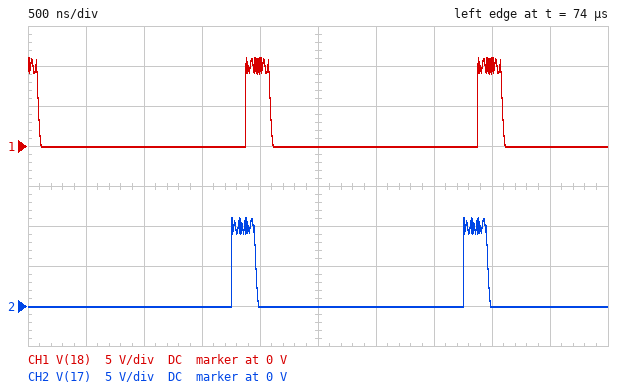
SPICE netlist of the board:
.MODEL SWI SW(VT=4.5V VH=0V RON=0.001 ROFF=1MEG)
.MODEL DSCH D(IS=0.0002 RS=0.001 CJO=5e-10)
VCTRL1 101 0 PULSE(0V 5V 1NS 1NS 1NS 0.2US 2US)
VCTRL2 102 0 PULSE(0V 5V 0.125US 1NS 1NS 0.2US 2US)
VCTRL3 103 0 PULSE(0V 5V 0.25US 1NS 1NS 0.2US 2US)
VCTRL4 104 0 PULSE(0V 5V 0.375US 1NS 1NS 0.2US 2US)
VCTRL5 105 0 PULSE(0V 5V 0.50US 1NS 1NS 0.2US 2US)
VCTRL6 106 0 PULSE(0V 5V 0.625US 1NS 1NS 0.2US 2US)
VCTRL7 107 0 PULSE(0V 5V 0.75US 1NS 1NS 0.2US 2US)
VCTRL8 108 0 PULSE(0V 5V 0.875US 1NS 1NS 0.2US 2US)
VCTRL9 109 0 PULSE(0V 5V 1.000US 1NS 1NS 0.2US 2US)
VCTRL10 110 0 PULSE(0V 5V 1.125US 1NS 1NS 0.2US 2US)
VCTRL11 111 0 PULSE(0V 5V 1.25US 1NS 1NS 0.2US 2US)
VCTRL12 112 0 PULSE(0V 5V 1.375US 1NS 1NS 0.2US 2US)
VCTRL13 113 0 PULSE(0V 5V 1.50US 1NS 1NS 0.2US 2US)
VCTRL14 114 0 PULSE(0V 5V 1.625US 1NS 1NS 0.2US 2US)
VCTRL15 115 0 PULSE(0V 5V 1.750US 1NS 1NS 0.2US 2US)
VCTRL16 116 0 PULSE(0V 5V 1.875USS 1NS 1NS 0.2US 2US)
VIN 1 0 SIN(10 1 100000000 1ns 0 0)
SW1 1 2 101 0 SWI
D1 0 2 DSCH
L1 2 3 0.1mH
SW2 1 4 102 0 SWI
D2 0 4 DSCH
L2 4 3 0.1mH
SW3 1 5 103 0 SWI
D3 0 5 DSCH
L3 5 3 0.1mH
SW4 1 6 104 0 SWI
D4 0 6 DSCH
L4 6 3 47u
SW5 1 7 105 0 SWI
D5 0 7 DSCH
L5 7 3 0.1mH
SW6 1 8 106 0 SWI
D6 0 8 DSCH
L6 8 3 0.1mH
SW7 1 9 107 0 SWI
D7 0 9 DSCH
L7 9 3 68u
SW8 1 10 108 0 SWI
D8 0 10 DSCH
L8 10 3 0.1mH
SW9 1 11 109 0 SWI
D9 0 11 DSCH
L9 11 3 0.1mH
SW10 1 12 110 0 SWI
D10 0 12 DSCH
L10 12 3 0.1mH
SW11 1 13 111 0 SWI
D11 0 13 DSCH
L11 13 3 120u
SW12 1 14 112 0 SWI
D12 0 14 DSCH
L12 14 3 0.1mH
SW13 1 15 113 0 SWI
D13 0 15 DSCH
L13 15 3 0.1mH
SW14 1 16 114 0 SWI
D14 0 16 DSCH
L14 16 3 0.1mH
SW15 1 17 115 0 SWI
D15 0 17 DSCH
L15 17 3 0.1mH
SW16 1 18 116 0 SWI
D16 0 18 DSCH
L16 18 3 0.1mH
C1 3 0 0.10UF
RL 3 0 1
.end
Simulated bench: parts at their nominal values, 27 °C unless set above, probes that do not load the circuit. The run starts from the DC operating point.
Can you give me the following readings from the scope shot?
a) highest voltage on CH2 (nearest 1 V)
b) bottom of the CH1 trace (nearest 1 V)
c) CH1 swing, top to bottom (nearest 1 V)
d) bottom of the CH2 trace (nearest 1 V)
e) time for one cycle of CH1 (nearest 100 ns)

11 V
0 V
11 V
0 V
2.0 µs
